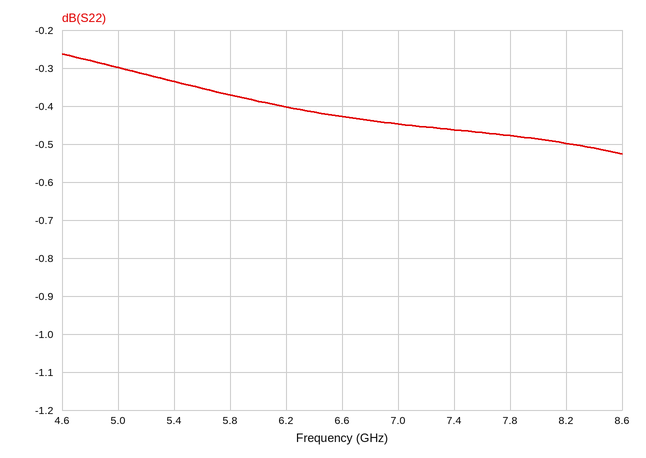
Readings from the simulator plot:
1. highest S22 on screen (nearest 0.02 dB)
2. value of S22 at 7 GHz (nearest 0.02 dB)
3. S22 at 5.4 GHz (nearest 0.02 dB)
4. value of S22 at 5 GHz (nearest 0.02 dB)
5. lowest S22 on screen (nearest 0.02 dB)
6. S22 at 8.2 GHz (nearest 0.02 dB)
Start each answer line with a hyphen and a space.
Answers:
- -0.26 dB
- -0.44 dB
- -0.34 dB
- -0.30 dB
- -0.52 dB
- -0.50 dB
